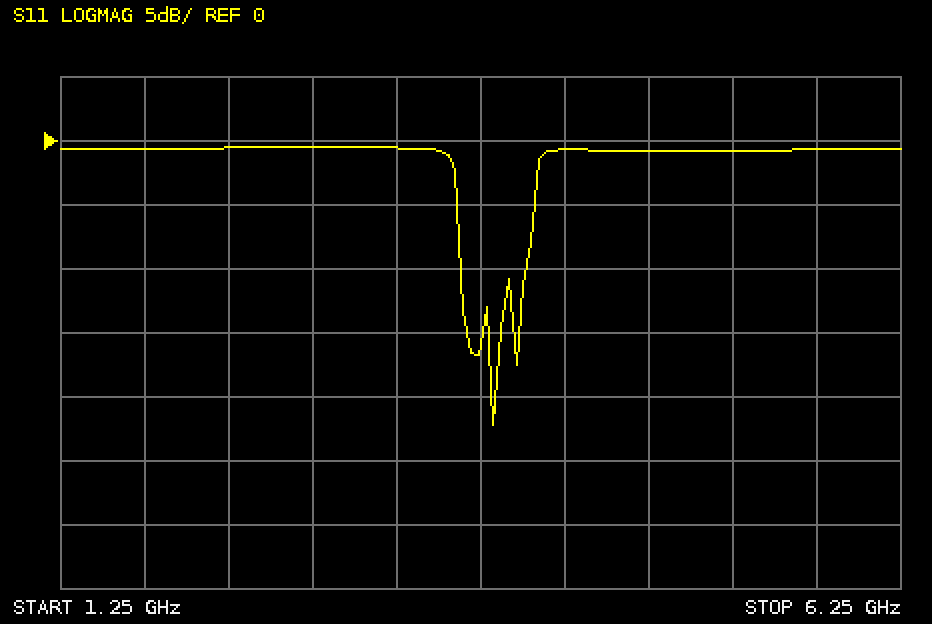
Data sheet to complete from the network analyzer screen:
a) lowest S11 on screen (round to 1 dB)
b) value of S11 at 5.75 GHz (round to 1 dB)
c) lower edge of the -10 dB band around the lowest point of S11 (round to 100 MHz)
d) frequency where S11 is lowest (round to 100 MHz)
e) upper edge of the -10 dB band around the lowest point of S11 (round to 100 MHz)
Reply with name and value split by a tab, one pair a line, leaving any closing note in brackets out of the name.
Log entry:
lowest S11 on screen	-22 dB
value of S11 at 5.75 GHz	-1 dB
lower edge of the -10 dB band around the lowest point of S11	3.6 GHz
frequency where S11 is lowest	3.8 GHz
upper edge of the -10 dB band around the lowest point of S11	4.0 GHz
